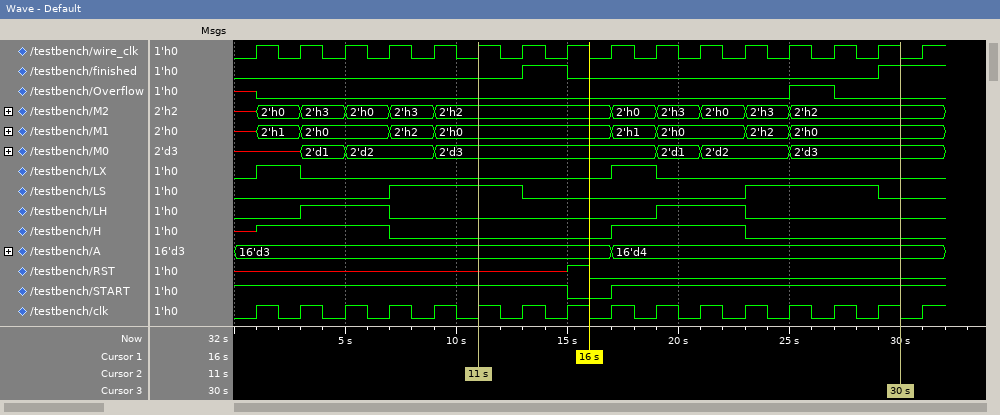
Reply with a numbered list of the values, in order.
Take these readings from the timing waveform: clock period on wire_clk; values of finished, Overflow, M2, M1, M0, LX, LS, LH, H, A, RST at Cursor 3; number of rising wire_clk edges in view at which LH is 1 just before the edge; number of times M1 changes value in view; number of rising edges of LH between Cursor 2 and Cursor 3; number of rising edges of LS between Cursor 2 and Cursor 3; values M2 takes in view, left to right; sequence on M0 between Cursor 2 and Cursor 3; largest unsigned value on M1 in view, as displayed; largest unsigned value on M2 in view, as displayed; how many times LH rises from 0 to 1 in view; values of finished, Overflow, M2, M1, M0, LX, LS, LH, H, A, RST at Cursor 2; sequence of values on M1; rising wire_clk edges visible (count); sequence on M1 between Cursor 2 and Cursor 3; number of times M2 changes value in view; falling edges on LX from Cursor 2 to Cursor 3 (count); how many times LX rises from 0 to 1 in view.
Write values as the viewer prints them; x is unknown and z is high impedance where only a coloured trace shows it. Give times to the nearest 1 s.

1. 2 s
2. finished=1, Overflow=0, M2=2'h2, M1=2'h0, M0=2'd3, LX=0, LS=0, LH=0, H=0, A=16'd4, RST=0
3. 4
4. 8
5. 1
6. 1
7. x, 2'h0, 2'h3, 2'h0, 2'h3, 2'h2, 2'h0, 2'h3, 2'h0, 2'h3, 2'h2
8. 2'd3, 2'd1, 2'd2, 2'd3
9. 2'h2
10. 2'h3
11. 2
12. finished=0, Overflow=0, M2=2'h2, M1=2'h0, M0=2'd3, LX=0, LS=1, LH=0, H=0, A=16'd3, RST=x
13. x, 2'h1, 2'h0, 2'h2, 2'h0, 2'h1, 2'h0, 2'h2, 2'h0
14. 16
15. 2'h0, 2'h1, 2'h0, 2'h2, 2'h0
16. 10
17. 1
18. 2
